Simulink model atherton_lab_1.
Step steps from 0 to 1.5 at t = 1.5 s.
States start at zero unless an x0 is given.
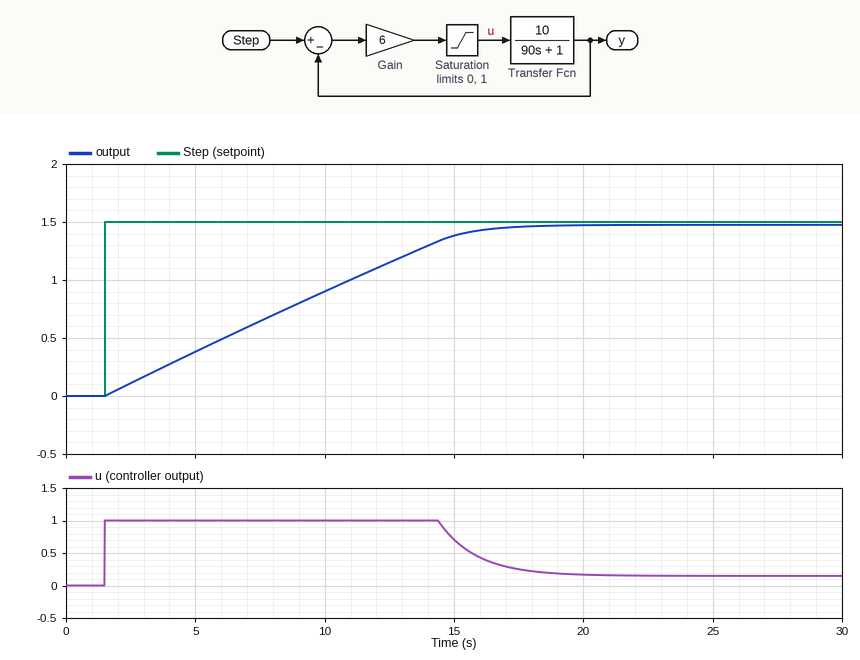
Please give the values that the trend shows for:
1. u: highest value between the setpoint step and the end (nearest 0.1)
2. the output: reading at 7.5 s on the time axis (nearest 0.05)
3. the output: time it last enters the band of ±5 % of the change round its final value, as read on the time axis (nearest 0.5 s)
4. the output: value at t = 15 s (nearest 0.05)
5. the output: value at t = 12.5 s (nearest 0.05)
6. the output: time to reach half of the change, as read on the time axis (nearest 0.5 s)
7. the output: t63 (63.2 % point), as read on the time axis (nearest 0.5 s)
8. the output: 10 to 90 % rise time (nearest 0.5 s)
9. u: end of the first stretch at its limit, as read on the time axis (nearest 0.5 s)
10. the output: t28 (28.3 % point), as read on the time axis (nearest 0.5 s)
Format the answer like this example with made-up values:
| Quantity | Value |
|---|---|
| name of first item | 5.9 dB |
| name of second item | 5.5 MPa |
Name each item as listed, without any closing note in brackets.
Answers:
| Quantity | Value |
|---|---|
| u: highest value between the setpoint step and the end | 1.0 |
| the output: reading at 7.5 s on the time axis | 0.65 |
| the output: time it last enters the band of ±5 % of the change round its final value, as read on the time axis | 15.5 s |
| the output: value at t = 15 s | 1.40 |
| the output: value at t = 12.5 s | 1.15 |
| the output: time to reach half of the change, as read on the time axis | 8.5 s |
| the output: t63 (63.2 % point), as read on the time axis | 10.5 s |
| the output: 10 to 90 % rise time | 11.5 s |
| u: end of the first stretch at its limit, as read on the time axis | 14.5 s |
| the output: t28 (28.3 % point), as read on the time axis | 5.5 s |
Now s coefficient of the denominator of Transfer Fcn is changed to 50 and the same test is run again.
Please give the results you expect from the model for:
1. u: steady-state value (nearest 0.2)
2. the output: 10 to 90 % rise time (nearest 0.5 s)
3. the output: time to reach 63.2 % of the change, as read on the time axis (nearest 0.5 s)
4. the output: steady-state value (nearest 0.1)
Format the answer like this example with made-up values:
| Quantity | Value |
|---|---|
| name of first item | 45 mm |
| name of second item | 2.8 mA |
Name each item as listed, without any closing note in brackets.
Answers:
| Quantity | Value |
|---|---|
| u: steady-state value | 0.2 |
| the output: 10 to 90 % rise time | 6.5 s |
| the output: time to reach 63.2 % of the change, as read on the time axis | 6.5 s |
| the output: steady-state value | 1.5 |
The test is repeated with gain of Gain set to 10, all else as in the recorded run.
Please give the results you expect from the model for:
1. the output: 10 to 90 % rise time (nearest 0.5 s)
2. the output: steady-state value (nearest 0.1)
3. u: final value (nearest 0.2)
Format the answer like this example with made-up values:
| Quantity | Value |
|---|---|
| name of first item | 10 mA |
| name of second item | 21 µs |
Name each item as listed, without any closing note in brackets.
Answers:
| Quantity | Value |
|---|---|
| the output: 10 to 90 % rise time | 11.5 s |
| the output: steady-state value | 1.5 |
| u: final value | 0.2 |
